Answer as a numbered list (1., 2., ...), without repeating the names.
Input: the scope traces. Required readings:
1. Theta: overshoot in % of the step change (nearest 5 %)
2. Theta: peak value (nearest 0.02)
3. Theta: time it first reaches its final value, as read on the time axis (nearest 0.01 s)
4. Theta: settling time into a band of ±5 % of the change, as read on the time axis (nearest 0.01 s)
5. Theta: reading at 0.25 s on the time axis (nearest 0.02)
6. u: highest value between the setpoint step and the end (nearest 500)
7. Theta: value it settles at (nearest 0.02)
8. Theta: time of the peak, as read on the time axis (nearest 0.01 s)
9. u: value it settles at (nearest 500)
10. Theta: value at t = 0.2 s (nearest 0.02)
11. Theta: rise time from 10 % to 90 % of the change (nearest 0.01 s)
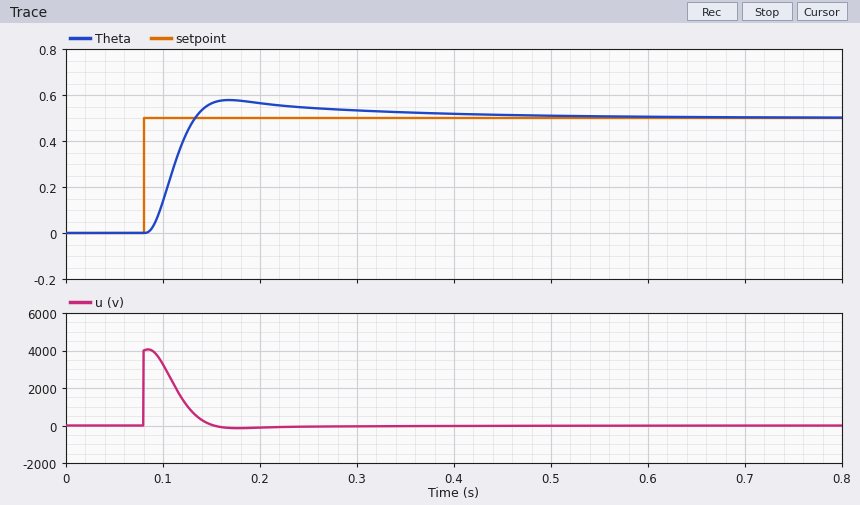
1. 15 %
2. 0.58
3. 0.13 s
4. 0.35 s
5. 0.54
6. 4000
7. 0.50
8. 0.17 s
9. 0
10. 0.56
11. 0.03 s
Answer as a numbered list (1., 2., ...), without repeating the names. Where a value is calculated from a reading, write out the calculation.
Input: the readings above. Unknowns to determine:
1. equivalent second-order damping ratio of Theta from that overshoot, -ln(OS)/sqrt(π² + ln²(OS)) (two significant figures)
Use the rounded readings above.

1. ln(0.15) = -1.897; 1.897 / sqrt(9.870 + 3.599) = 0.52
